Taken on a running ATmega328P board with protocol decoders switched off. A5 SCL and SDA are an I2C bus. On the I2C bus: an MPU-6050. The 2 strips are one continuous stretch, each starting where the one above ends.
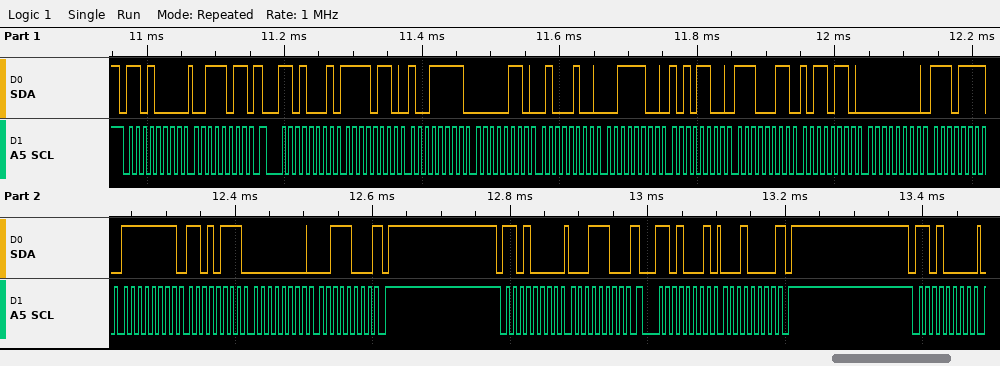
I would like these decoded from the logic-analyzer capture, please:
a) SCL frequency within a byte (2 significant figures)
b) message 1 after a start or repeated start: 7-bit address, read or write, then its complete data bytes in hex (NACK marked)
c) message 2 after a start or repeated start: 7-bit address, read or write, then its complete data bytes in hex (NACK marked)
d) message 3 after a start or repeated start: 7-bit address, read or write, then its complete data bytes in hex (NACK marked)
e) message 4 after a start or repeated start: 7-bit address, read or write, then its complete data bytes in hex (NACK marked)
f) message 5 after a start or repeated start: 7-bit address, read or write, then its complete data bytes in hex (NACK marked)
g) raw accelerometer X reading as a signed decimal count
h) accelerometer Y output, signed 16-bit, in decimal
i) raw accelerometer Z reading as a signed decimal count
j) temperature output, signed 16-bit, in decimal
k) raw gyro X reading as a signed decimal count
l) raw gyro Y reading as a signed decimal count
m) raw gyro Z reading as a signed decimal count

100 kHz
0x68 write: 3B
0x68 read: F6 9F 06 44 3C AC E3 B6 00 EF FF D7 00 38 NACK
0x68 write: 1C
0x68 read: 10 NACK
0x68 write
-2401
1604
15532
-7242
239
-41
56
